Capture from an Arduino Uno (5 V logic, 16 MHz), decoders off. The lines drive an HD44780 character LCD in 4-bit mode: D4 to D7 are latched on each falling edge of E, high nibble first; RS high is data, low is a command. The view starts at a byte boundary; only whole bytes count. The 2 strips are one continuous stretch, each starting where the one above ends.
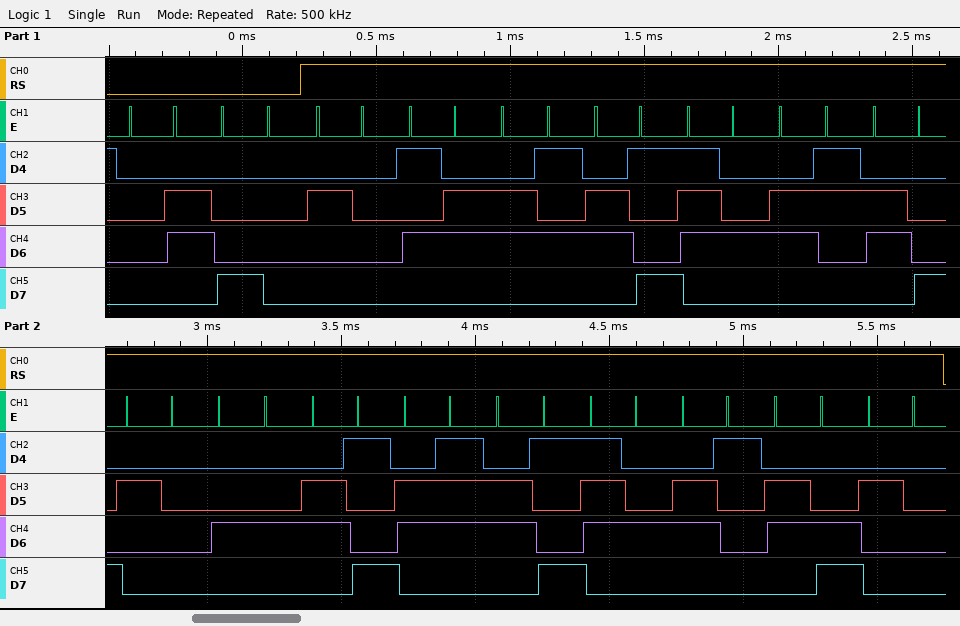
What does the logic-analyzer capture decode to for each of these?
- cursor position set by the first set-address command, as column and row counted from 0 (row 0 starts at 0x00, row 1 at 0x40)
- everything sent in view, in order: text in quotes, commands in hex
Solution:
column 0, row 0
0x06 0x80 " Veitch Digital "
